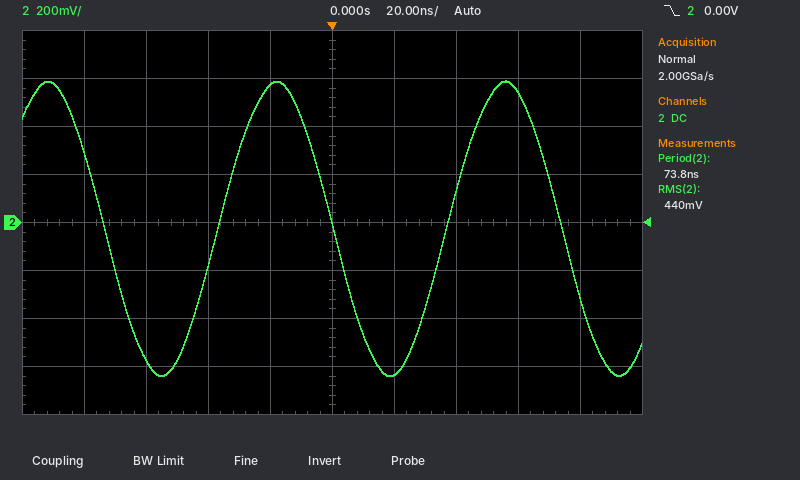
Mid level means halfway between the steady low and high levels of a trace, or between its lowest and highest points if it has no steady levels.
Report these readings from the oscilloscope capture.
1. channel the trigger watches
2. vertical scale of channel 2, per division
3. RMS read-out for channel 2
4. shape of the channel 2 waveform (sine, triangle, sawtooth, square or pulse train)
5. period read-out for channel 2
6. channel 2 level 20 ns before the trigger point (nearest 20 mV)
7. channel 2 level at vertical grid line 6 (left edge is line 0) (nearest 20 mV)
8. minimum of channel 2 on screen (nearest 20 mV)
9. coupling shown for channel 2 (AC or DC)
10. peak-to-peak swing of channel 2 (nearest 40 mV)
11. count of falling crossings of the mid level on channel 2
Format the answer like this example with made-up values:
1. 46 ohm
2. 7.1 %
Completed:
1. channel 2
2. 200 mV
3. 440 mV
4. sine
5. 73.8 ns
6. 580 mV
7. -640 mV
8. -640 mV
9. DC
10. 1.24 V
11. 3
